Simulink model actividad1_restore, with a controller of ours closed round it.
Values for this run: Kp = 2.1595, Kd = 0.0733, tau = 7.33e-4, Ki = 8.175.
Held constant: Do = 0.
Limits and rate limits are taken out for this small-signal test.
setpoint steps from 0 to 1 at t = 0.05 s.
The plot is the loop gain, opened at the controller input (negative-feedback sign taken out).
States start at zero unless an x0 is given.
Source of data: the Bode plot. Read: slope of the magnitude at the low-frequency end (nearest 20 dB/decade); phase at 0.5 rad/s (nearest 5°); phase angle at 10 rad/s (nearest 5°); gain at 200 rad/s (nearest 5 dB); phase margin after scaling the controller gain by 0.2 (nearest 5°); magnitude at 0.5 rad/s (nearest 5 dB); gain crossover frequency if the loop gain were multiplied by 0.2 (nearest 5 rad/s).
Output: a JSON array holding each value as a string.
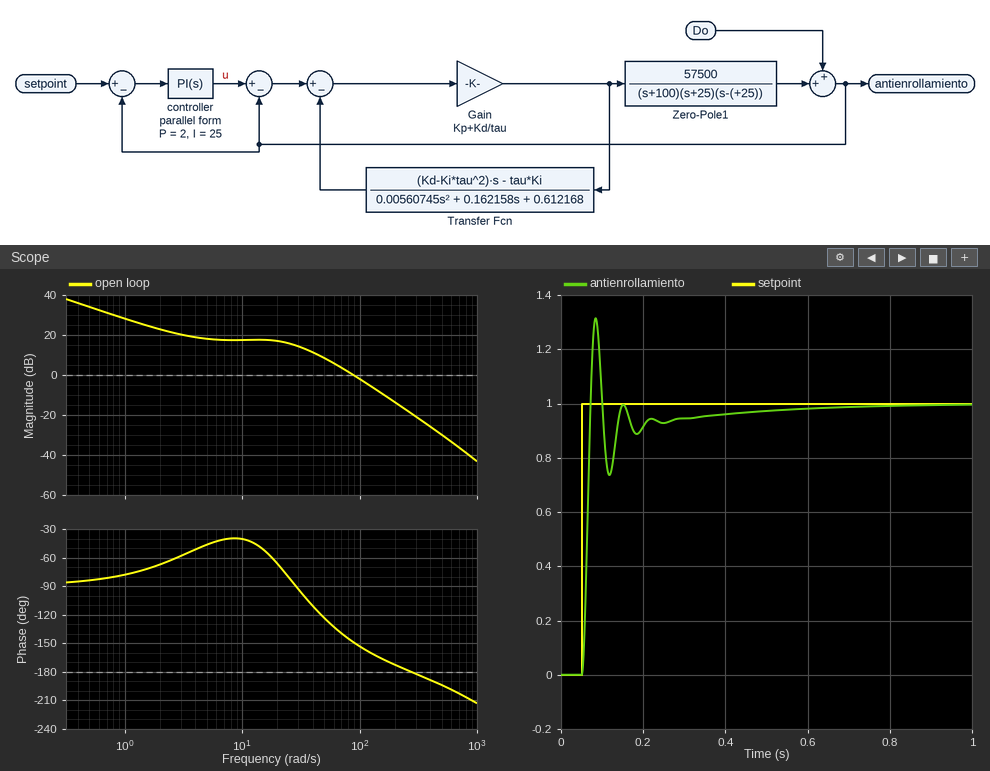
["-20 dB/decade", "-85°", "-40°", "-15 dB", "85°", "35 dB", "30 rad/s"]
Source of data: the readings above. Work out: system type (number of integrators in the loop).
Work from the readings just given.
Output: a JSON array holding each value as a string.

["1"]
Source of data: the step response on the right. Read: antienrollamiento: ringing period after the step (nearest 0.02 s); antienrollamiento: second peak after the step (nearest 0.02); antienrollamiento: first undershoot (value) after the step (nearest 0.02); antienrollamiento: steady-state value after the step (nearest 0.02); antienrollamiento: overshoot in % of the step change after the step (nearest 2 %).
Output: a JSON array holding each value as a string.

["0.06 s", "1.00", "0.74", "1.00", "32 %"]
